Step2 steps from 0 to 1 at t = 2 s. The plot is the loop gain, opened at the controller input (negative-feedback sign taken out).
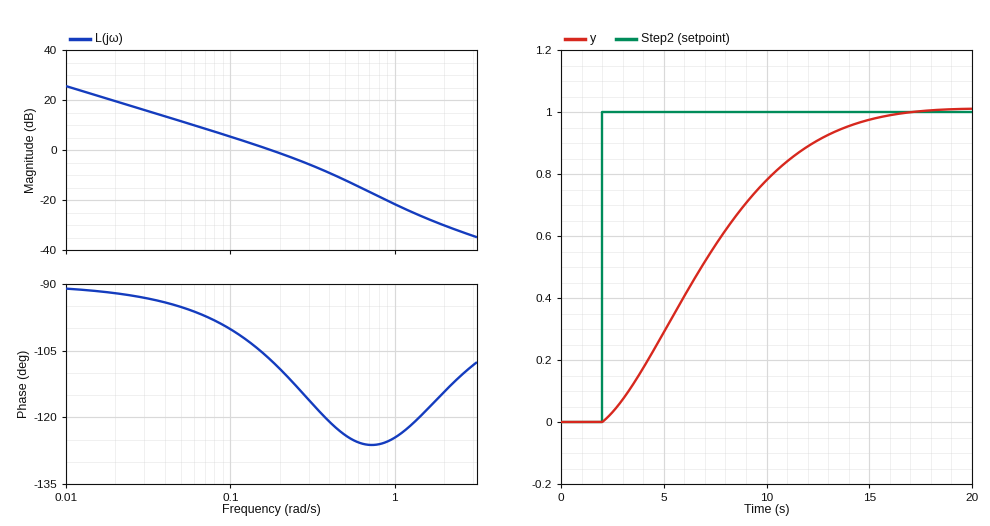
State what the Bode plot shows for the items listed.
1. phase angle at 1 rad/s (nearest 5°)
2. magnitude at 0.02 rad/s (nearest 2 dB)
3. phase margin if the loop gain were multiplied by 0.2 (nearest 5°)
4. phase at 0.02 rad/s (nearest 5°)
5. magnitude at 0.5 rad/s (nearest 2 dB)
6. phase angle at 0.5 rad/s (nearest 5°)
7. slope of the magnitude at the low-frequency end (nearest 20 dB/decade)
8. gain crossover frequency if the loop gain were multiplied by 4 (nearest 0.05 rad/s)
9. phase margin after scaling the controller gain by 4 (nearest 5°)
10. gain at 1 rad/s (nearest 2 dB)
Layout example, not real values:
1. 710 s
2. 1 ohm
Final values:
1. -125°
2. 20 dB
3. 85°
4. -90°
5. -12 dB
6. -125°
7. -20 dB/decade
8. 0.50 rad/s
9. 55°
10. -22 dB
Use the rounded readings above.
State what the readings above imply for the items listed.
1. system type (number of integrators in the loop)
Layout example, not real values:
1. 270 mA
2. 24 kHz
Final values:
1. 1
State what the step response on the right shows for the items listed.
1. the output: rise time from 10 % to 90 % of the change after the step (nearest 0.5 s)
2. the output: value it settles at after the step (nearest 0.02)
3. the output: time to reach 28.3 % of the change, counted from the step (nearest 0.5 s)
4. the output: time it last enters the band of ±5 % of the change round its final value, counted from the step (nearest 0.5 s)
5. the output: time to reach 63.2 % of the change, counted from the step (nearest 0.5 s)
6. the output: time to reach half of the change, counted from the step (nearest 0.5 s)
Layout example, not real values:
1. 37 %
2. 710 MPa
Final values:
1. 9.0 s
2. 1.00
3. 3.0 s
4. 12.0 s
5. 6.0 s
6. 5.0 s
